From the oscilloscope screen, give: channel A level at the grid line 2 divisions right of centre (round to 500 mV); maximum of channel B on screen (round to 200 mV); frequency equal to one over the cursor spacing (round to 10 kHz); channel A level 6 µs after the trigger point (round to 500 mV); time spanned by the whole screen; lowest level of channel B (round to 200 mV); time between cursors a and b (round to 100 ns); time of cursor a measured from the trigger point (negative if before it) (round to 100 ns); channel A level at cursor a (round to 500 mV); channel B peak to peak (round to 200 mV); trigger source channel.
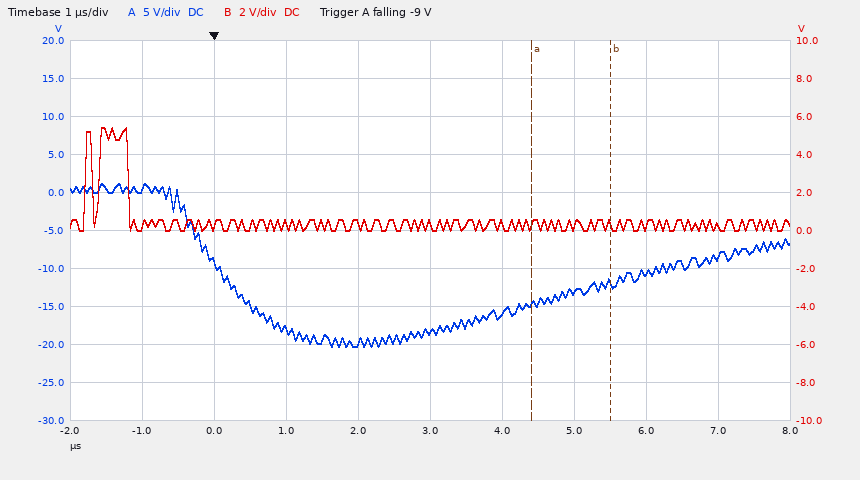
-13.0 V
5.4 V
910 kHz
-10.5 V
10 µs
0.0 V
1.1 µs
+4.4 µs
-14.5 V
5.4 V
channel A
